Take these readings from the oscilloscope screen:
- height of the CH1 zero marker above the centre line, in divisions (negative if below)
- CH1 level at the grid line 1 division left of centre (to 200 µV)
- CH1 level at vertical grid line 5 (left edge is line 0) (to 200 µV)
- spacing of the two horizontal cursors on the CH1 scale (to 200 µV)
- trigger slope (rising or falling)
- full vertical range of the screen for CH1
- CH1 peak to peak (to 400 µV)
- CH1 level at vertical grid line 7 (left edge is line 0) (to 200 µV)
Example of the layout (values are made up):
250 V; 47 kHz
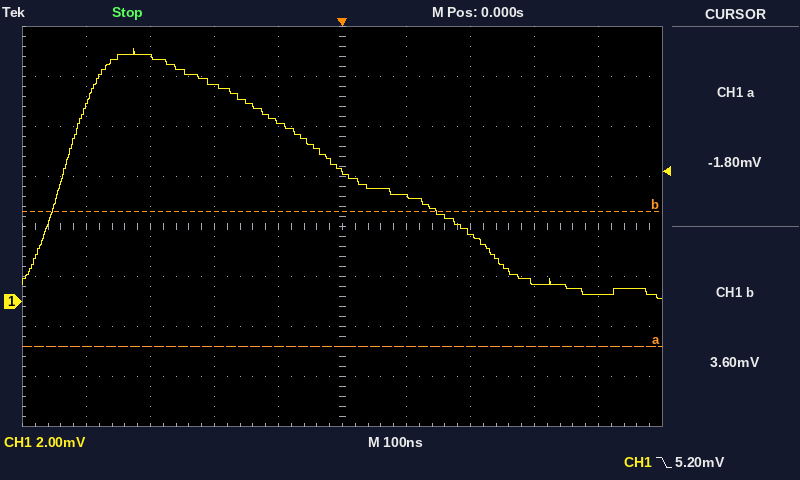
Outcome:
-1.5 div; 7.2 mV; 5.2 mV; 5.4 mV; falling; 16 mV; 10.0 mV; 2.8 mV
